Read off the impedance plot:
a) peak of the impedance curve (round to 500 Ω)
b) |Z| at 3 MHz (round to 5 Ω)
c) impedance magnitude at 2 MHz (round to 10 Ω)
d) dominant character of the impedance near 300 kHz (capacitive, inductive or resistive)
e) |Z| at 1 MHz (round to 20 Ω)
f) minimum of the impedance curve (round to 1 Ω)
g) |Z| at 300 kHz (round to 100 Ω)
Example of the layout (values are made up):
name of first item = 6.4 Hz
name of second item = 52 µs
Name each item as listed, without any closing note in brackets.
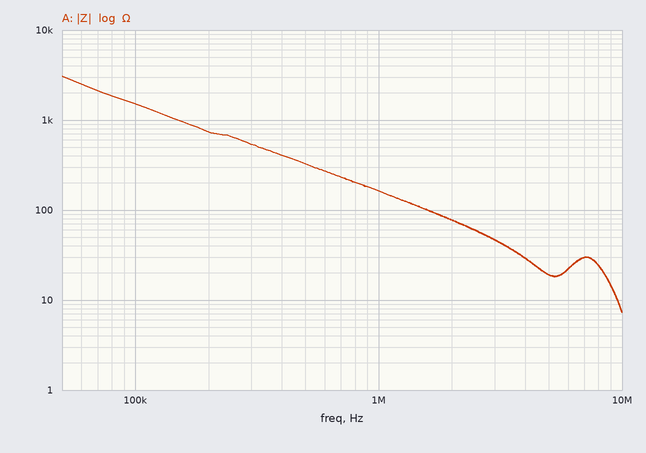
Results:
peak of the impedance curve = 3.0 kΩ
|Z| at 3 MHz = 45 Ω
impedance magnitude at 2 MHz = 80 Ω
dominant character of the impedance near 300 kHz = capacitive
|Z| at 1 MHz = 160 Ω
minimum of the impedance curve = 7 Ω
|Z| at 300 kHz = 500 Ω
